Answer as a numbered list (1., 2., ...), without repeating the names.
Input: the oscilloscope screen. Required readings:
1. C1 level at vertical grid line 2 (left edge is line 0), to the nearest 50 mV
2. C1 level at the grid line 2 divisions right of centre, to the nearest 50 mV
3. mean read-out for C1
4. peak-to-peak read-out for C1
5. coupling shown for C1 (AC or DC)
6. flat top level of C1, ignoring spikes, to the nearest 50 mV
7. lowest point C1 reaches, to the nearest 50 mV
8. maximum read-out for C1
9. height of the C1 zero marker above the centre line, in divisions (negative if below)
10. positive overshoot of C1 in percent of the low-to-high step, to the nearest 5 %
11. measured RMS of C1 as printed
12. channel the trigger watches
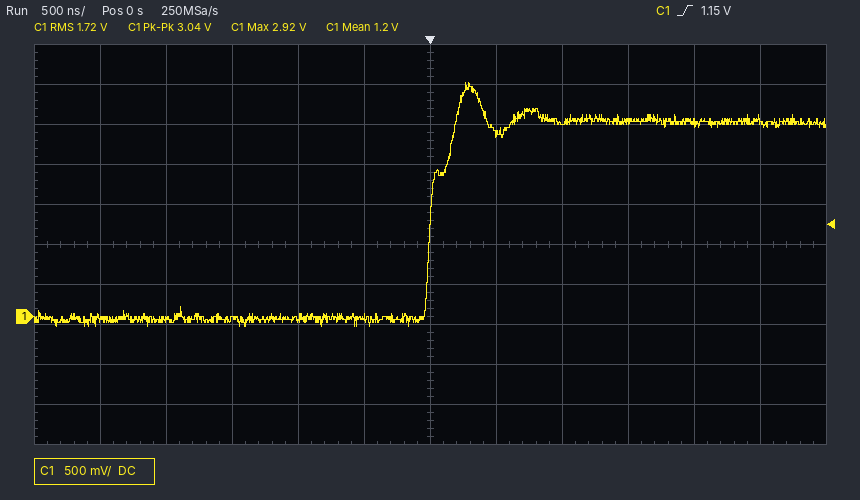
1. -50 mV
2. 2.40 V
3. 1.2 V
4. 3.04 V
5. DC
6. 2.45 V
7. -100 mV
8. 2.92 V
9. -1.8 div
10. 20 %
11. 1.72 V
12. C1
